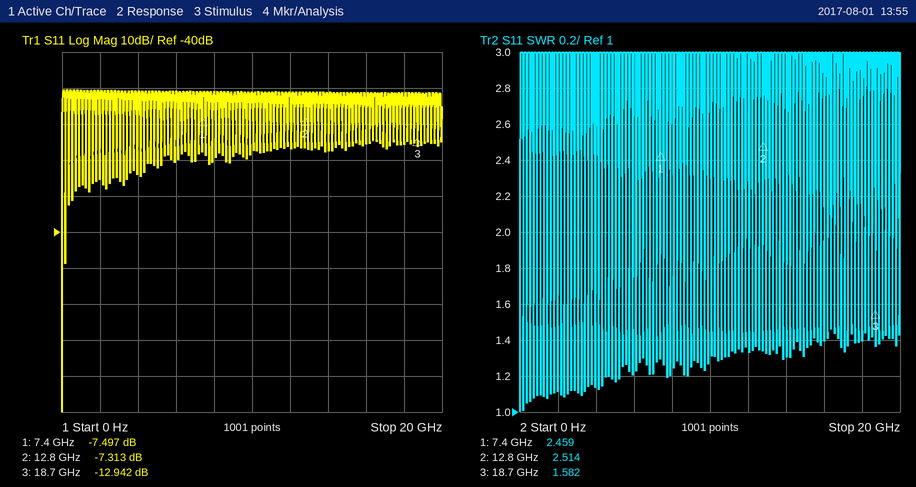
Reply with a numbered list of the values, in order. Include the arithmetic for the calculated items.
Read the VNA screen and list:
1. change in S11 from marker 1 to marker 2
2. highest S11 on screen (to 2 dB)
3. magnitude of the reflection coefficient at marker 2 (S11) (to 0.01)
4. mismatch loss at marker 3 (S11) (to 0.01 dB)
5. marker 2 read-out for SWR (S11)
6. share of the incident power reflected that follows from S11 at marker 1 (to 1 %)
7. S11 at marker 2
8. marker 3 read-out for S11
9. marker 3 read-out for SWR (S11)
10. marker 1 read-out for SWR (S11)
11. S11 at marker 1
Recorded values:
1. -7.313 − (-7.497) = 0.184 dB
2. 0 dB
3. 10^(-7.313/20) ≈ 0.43
4. −10 log10(1 − 10^(-12.942/10)) ≈ 0.23 dB
5. 2.514
6. 10^(-7.497/10) ≈ 18 %
7. -7.313 dB
8. -12.942 dB
9. 1.582
10. 2.459
11. -7.497 dB
